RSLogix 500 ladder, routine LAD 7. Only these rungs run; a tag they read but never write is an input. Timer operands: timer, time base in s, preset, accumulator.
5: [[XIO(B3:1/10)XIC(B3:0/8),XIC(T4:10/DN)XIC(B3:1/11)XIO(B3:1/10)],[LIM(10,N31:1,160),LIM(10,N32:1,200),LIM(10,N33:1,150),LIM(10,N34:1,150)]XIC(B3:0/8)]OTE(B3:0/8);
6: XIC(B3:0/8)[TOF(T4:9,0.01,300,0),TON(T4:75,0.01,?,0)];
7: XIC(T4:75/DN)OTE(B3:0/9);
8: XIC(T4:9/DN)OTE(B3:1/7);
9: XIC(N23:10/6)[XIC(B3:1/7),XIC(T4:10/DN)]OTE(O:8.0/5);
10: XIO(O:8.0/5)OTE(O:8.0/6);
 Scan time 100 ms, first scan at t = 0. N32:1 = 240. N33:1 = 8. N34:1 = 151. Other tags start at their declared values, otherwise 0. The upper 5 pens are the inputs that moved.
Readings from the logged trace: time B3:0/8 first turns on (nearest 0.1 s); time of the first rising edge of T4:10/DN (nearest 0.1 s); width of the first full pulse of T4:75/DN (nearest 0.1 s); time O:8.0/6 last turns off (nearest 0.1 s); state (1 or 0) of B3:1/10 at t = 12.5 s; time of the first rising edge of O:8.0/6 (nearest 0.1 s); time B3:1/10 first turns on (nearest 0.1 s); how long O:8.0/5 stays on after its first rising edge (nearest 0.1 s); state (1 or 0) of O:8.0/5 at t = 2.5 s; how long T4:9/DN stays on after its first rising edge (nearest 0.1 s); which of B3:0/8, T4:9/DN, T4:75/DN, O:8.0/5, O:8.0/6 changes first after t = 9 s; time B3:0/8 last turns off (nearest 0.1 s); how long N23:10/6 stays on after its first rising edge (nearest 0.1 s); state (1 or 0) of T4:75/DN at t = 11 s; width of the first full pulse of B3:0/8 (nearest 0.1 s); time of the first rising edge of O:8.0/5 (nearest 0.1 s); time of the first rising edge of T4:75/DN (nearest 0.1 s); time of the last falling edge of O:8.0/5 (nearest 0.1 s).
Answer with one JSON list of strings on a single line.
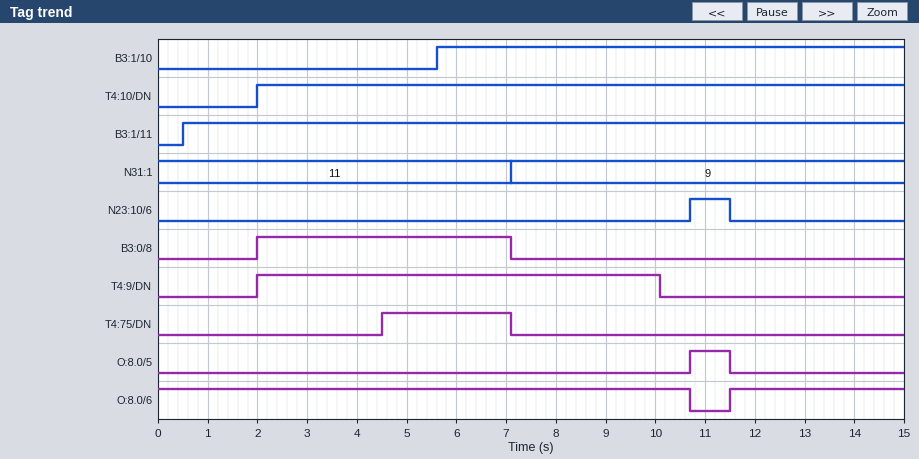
["2.0 s", "2.0 s", "2.6 s", "10.7 s", "1", "11.5 s", "5.6 s", "0.8 s", "0", "8.1 s", "T4:9/DN", "7.1 s", "0.8 s", "0", "5.1 s", "10.7 s", "4.5 s", "11.5 s"]
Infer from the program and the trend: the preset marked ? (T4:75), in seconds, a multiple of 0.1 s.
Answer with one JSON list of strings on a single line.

["2.5 s"]
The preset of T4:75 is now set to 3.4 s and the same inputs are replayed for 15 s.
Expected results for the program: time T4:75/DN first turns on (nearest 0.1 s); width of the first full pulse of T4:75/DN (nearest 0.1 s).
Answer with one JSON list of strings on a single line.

["5.4 s", "1.7 s"]
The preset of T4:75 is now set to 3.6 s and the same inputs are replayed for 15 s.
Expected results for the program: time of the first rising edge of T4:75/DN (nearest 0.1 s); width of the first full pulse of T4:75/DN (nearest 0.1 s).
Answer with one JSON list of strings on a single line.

["5.6 s", "1.5 s"]
